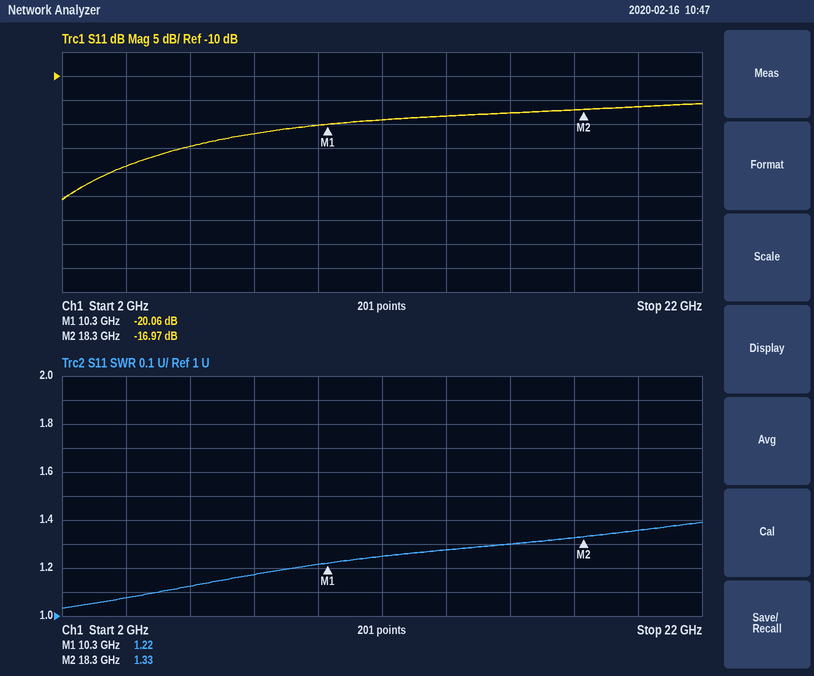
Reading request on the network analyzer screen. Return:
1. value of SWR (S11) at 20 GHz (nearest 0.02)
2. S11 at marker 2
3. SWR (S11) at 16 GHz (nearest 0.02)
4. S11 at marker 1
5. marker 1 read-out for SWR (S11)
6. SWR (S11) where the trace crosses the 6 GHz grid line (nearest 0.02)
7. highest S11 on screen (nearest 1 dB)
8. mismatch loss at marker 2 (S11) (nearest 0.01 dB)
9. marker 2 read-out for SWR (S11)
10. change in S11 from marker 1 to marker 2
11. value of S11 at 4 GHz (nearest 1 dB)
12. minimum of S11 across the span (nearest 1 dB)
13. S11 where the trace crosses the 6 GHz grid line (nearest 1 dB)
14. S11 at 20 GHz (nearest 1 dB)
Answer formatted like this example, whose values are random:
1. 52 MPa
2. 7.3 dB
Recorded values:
1. 1.36
2. -16.97 dB
3. 1.30
4. -20.06 dB
5. 1.22
6. 1.12
7. -16 dB
8. 0.09 dB
9. 1.33
10. 3.09 dB
11. -29 dB
12. -36 dB
13. -25 dB
14. -16 dB
